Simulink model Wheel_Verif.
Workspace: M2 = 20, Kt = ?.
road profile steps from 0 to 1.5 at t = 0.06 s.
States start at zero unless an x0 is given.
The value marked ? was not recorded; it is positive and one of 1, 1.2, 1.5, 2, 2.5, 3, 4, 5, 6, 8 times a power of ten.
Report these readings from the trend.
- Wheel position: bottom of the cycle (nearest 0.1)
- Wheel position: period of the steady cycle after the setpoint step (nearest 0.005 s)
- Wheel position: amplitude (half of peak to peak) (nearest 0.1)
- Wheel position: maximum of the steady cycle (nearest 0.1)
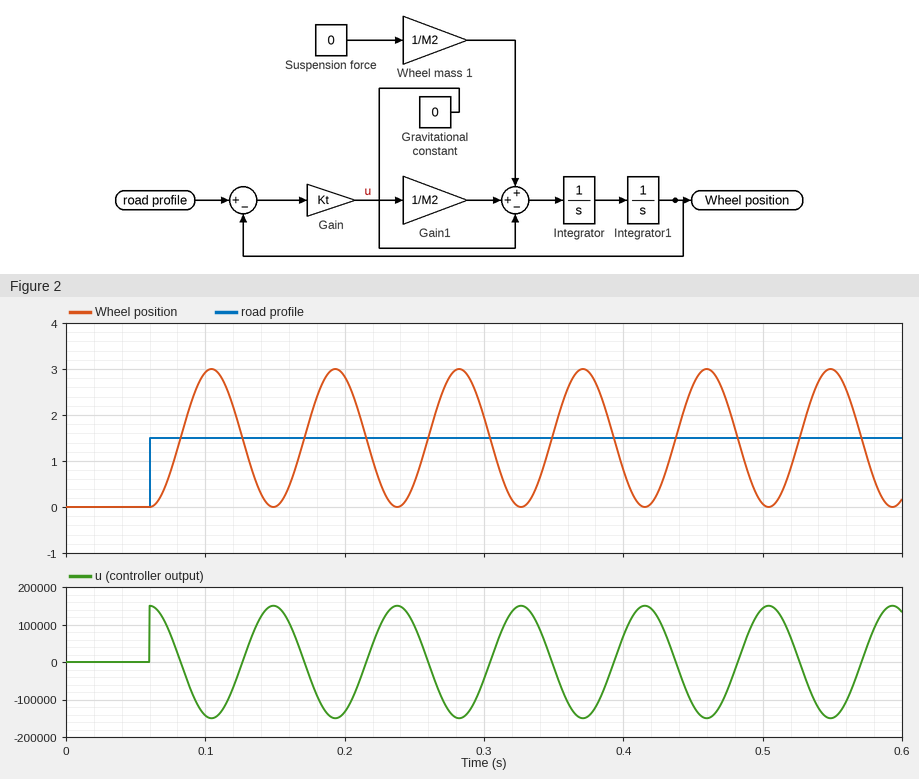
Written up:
0.0
0.090 s
1.5
3.0
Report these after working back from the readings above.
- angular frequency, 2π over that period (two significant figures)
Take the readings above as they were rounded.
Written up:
70 rad/s
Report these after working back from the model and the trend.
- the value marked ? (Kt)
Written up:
100000
